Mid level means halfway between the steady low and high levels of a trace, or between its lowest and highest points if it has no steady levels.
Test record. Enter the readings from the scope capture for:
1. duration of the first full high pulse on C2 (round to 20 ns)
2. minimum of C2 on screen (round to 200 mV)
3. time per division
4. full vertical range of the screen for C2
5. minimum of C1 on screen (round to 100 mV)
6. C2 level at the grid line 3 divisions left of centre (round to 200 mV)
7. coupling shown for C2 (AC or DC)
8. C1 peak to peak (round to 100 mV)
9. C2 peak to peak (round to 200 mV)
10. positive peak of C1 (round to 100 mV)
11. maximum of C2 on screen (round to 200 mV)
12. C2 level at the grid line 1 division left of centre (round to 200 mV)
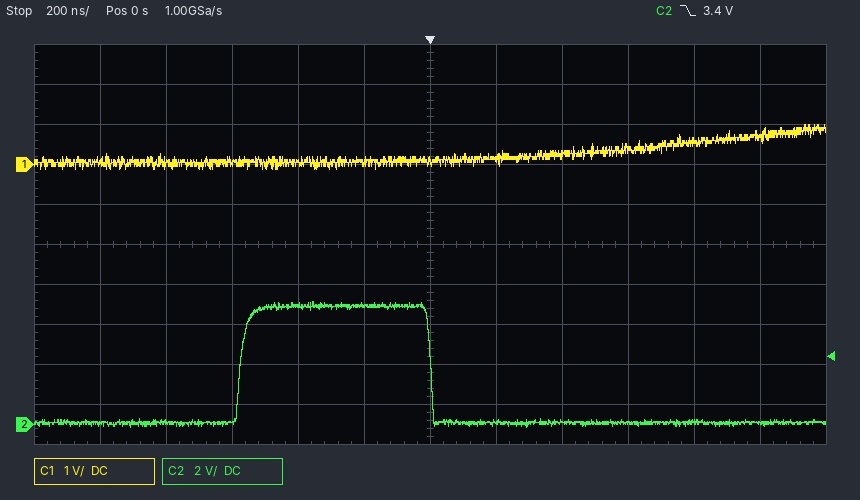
580 ns
-200 mV
200 ns
20 V
-100 mV
200 mV
DC
1.1 V
6.4 V
1.0 V
6.2 V
6.0 V
